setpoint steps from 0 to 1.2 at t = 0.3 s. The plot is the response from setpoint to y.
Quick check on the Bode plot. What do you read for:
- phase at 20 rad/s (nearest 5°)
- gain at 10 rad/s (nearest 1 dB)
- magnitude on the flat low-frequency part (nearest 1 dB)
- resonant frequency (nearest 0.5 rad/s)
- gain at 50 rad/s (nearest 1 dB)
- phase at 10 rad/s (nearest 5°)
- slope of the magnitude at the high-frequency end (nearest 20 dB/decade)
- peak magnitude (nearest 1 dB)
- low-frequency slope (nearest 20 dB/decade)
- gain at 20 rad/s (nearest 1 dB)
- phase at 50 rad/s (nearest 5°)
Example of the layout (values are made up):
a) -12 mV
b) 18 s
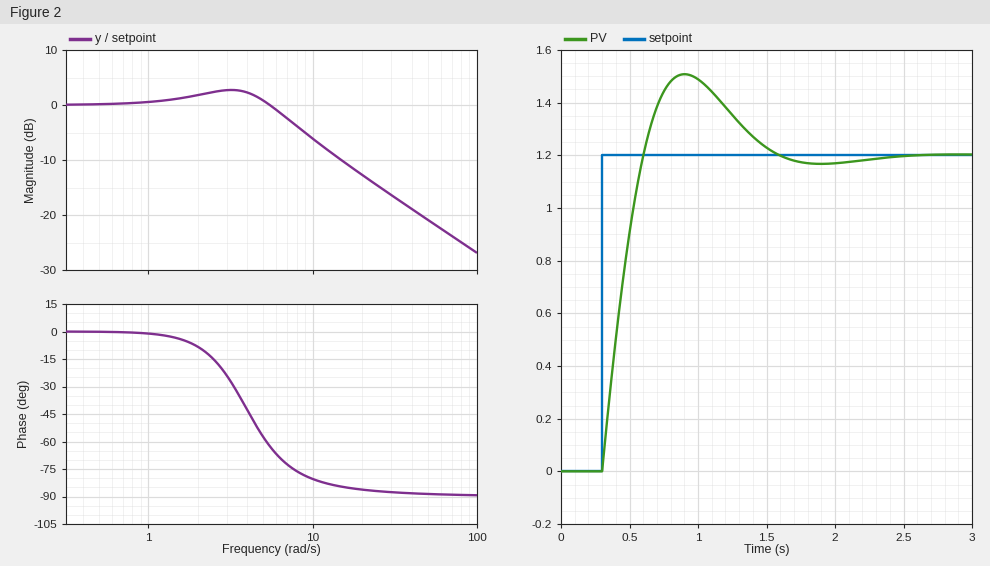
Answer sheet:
a) -85°
b) -6 dB
c) 0 dB
d) 3.0 rad/s
e) -21 dB
f) -80°
g) -20 dB/decade
h) 3 dB
i) 0 dB/decade
j) -13 dB
k) -90°
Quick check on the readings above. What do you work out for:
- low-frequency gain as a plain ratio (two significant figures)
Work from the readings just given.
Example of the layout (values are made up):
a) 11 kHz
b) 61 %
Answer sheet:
a) 1.0
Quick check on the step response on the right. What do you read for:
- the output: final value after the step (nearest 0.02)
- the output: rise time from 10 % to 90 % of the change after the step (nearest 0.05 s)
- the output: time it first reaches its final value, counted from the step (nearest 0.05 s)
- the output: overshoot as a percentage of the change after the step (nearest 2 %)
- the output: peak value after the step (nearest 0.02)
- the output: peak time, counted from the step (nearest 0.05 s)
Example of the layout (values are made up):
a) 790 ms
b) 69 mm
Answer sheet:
a) 1.20
b) 0.25 s
c) 0.30 s
d) 26 %
e) 1.50
f) 0.60 s
